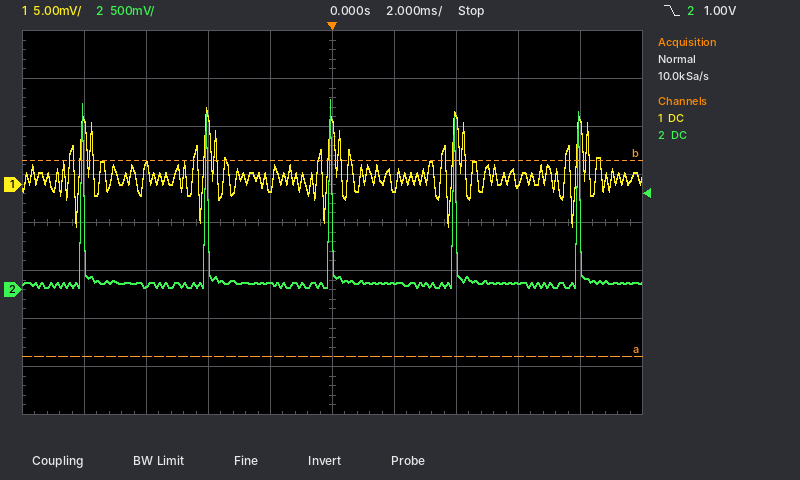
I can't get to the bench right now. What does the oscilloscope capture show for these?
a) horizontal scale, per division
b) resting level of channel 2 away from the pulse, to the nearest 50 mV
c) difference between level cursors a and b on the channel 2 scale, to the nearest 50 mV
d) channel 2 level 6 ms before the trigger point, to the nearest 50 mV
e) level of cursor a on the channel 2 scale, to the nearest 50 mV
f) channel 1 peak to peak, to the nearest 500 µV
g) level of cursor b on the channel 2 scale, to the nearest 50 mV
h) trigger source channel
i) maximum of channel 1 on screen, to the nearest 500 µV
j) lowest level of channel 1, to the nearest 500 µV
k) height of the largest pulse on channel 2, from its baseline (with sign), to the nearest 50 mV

2 ms
50 mV
2.05 V
50 mV
-700 mV
12.5 mV
1.35 V
channel 2
8.0 mV
-4.5 mV
+1.90 V
